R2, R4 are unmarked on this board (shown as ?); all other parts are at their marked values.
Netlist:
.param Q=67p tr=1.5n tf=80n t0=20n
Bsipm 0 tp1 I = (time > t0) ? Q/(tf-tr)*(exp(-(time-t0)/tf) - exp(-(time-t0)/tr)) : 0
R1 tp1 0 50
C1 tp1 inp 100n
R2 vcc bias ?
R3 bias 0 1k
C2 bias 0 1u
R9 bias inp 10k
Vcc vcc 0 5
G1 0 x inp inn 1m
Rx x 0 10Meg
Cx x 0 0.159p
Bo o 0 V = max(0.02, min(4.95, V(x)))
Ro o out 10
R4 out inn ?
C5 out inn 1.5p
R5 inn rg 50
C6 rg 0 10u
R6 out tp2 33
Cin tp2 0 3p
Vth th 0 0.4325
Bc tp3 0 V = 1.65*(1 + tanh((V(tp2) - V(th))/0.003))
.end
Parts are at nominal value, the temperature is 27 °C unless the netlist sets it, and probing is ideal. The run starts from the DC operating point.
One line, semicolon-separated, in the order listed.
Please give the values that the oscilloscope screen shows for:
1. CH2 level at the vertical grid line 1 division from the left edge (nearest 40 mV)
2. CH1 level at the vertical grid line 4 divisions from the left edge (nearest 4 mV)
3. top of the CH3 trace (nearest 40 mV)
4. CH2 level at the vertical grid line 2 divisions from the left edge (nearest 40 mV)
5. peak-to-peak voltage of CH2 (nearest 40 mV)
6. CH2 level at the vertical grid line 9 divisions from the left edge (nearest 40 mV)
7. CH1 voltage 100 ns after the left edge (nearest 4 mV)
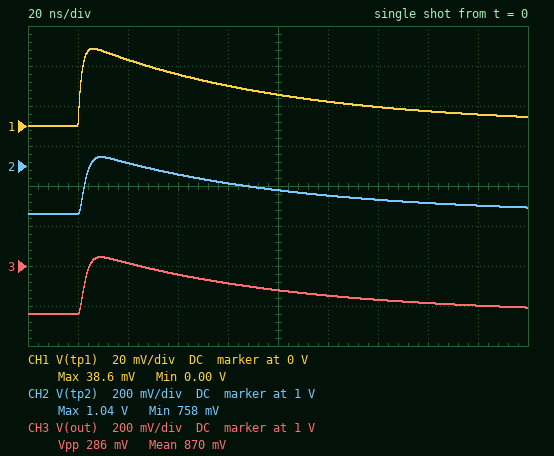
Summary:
760 mV; 20 mV; 1.04 V; 1.00 V; 280 mV; 800 mV; 16 mV
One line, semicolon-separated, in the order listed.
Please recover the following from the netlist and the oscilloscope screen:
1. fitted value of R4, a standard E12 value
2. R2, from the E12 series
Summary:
330 Ω; 5.6 kΩ
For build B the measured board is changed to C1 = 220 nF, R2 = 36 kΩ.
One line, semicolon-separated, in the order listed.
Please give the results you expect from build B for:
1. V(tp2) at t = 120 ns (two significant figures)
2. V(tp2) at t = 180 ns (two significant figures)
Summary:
230 mV; 180 mV
